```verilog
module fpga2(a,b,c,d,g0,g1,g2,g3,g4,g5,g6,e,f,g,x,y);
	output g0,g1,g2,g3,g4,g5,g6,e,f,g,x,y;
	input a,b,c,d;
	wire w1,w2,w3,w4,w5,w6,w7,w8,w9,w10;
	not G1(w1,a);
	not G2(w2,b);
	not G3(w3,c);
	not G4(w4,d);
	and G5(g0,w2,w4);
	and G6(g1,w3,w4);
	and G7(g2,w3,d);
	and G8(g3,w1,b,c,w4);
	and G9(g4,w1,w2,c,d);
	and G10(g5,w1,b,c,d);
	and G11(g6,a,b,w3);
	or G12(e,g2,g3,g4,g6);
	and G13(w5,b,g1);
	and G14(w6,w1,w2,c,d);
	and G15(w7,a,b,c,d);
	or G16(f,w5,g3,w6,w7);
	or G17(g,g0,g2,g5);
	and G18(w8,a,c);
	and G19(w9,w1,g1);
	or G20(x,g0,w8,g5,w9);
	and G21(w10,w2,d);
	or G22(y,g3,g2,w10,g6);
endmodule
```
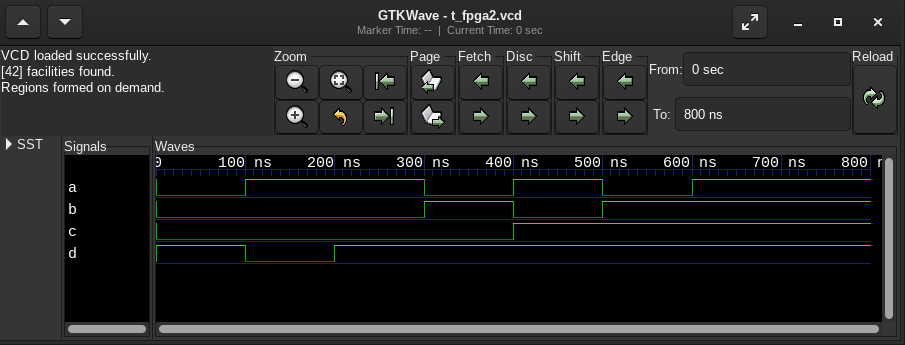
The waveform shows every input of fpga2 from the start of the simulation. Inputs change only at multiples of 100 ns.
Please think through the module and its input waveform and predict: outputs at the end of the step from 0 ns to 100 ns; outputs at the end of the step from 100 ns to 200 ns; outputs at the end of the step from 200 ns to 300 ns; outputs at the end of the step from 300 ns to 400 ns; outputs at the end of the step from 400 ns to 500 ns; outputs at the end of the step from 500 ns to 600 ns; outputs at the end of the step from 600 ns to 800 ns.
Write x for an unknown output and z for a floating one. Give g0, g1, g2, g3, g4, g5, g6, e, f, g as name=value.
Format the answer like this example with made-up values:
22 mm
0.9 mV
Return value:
g0=0, g1=0, g2=1, g3=0, g4=0, g5=0, g6=0, e=1, f=0, g=1
g0=1, g1=1, g2=0, g3=0, g4=0, g5=0, g6=0, e=0, f=0, g=1
g0=0, g1=0, g2=1, g3=0, g4=0, g5=0, g6=0, e=1, f=0, g=1
g0=0, g1=0, g2=1, g3=0, g4=0, g5=0, g6=0, e=1, f=0, g=1
g0=0, g1=0, g2=0, g3=0, g4=0, g5=0, g6=0, e=0, f=0, g=0
g0=0, g1=0, g2=0, g3=0, g4=0, g5=1, g6=0, e=0, f=0, g=1
g0=0, g1=0, g2=0, g3=0, g4=0, g5=0, g6=0, e=0, f=1, g=0
